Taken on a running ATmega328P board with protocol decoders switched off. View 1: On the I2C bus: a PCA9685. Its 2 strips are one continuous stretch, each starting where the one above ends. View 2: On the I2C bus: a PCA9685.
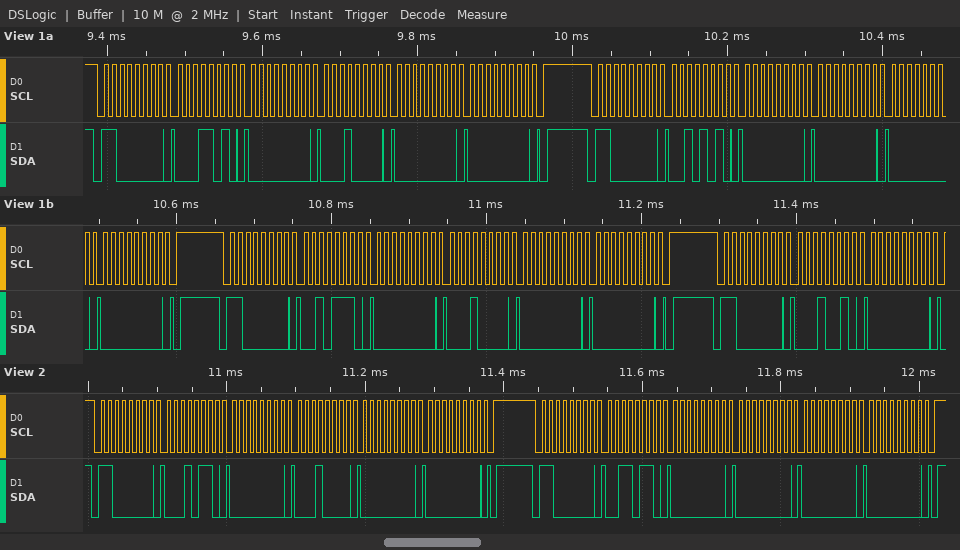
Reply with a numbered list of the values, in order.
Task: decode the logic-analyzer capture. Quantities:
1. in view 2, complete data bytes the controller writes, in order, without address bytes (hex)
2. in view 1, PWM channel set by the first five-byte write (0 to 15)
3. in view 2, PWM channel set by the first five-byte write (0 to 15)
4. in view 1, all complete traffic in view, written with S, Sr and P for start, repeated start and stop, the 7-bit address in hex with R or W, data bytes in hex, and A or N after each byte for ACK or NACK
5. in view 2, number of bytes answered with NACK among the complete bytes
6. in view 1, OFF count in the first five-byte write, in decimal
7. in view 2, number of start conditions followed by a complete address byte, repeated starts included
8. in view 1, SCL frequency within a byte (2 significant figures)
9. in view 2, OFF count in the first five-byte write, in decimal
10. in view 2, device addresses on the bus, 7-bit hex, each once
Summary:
1. 16 00 10 00 00 36 00 00 00 00
2. 5
3. 4
4. S 60W A 1A A 00 A 10 A 00 A 00 A P S 60W A 2A A 00 A 00 A 00 A 00 A P S 60W A 2E A 00 A 10 A 00 A 00 A P S 60W A 12 A 00 A
5. 0
6. 0
7. 2
8. 100 kHz
9. 0
10. 0x60
